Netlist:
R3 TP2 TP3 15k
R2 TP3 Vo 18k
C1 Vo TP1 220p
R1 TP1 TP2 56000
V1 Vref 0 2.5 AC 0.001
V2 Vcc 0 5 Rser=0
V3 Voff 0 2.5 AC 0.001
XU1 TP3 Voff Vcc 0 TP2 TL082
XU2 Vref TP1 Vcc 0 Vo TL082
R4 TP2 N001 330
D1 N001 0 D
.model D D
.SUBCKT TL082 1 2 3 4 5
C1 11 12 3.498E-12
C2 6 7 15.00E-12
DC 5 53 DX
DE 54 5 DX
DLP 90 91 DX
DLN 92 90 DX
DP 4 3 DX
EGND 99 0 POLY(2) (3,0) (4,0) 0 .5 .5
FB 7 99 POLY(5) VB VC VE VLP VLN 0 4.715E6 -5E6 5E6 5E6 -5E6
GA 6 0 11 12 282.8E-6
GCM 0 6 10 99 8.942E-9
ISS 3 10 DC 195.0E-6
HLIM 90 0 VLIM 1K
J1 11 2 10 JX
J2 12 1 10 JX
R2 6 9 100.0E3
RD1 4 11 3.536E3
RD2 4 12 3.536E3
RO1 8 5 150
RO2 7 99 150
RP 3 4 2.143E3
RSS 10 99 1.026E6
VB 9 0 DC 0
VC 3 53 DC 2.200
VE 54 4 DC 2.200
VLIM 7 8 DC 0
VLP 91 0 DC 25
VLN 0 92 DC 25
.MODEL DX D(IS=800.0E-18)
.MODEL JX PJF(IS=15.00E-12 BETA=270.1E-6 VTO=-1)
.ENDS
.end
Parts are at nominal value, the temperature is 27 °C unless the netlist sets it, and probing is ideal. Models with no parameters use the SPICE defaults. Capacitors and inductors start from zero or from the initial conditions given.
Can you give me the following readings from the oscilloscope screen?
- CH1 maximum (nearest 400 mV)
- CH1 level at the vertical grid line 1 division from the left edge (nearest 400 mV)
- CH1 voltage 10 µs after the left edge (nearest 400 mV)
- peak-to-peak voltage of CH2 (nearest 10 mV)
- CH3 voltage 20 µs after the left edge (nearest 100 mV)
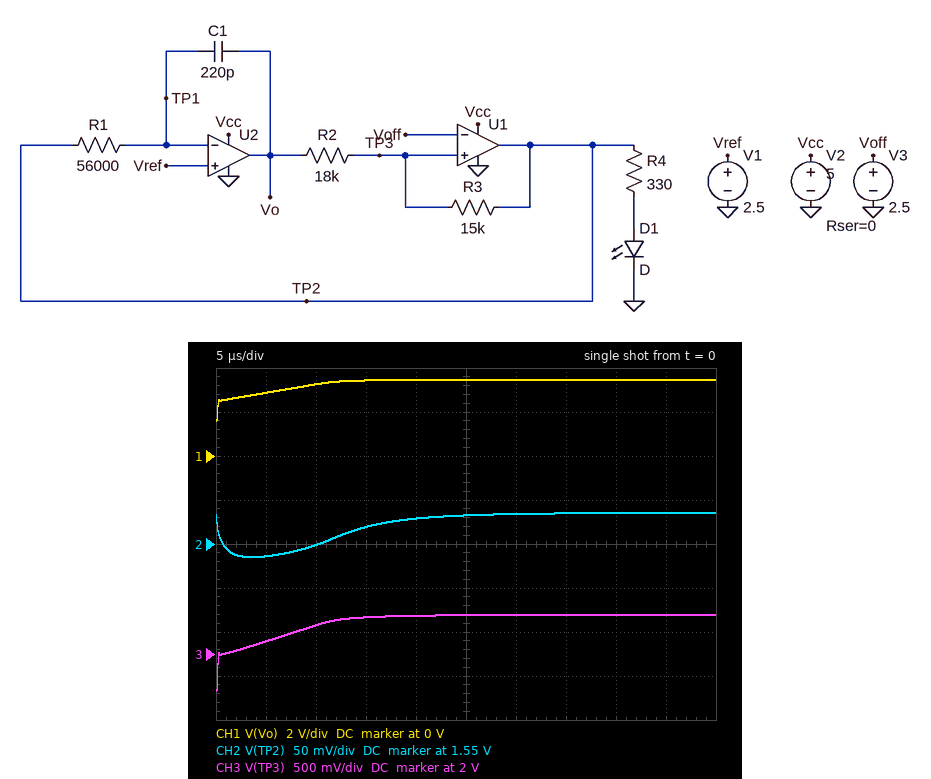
3.6 V
2.8 V
3.2 V
50 mV
2.4 V
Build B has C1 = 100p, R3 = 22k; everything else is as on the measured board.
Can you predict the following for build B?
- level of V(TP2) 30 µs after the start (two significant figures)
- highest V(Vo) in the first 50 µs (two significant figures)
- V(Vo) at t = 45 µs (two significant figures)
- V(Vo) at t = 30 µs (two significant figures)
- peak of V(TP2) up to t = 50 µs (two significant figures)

1.6 V
3.4 V
1.6 V
3.2 V
3.5 V
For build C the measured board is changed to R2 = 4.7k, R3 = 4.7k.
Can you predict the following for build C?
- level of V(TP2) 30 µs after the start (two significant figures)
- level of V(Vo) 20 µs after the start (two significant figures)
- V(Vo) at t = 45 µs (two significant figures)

3.5 V
3.2 V
1.6 V
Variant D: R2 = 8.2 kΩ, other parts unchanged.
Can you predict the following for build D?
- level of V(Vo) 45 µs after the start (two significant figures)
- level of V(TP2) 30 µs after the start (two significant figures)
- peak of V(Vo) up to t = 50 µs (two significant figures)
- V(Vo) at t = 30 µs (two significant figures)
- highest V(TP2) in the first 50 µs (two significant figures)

2.9 V
1.5 V
3.1 V
2.2 V
3.5 V
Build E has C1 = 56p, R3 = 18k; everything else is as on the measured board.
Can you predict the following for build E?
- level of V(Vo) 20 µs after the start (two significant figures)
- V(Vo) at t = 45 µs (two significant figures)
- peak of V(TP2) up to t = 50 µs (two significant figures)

1.5 V
1.6 V
3.5 V
